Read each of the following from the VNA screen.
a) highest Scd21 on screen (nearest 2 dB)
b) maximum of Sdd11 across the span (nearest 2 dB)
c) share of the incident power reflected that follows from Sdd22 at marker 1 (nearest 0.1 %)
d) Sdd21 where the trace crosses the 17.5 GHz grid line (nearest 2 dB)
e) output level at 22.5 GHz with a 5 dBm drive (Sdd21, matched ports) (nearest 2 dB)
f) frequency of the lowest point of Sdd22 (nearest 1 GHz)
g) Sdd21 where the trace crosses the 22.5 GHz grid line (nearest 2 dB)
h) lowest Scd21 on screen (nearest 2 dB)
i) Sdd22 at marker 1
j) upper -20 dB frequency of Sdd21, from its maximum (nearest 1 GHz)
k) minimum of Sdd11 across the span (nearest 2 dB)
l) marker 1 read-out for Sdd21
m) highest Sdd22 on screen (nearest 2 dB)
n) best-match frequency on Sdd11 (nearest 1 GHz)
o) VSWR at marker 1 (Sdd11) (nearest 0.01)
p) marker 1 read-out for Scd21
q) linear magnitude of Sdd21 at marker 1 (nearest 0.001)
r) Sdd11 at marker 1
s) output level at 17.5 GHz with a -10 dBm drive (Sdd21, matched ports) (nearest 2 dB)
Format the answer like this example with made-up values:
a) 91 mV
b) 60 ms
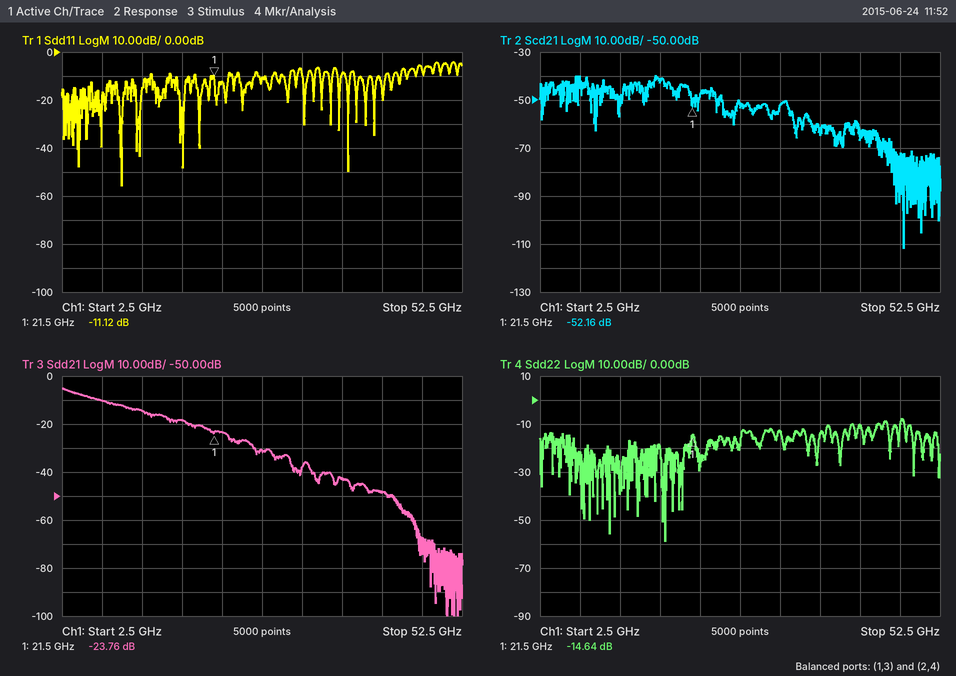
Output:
a) -40 dB
b) -4 dB
c) 3.4 %
d) -18 dB
e) -18 dBm
f) 18 GHz
g) -24 dB
h) -112 dB
i) -14.64 dB
j) 23 GHz
k) -56 dB
l) -23.76 dB
m) -8 dB
n) 10 GHz
o) 1.77
p) -52.16 dB
q) 0.065
r) -11.12 dB
s) -28 dBm
